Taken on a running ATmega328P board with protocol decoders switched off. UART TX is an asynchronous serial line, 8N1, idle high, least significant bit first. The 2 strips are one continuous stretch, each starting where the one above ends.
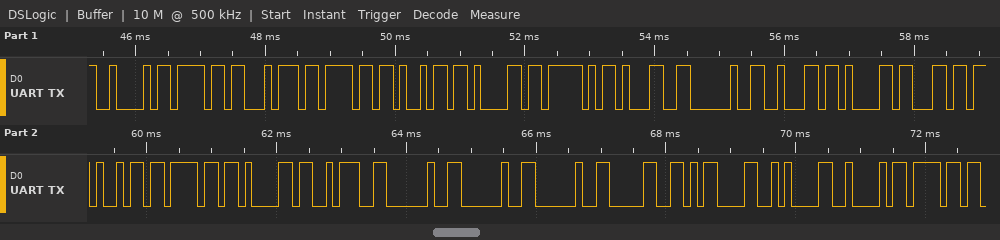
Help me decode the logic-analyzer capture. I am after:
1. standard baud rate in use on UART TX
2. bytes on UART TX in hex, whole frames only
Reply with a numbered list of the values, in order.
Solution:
1. 9600 baud
2. 42 6F 74 6F 69 61 5F 31 20 62 61 6C 69 6F 61 3A 20 20 20 30 0D 0A 42 6F
